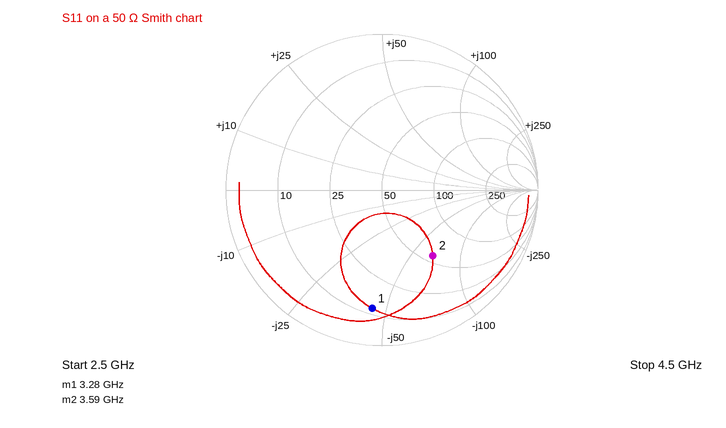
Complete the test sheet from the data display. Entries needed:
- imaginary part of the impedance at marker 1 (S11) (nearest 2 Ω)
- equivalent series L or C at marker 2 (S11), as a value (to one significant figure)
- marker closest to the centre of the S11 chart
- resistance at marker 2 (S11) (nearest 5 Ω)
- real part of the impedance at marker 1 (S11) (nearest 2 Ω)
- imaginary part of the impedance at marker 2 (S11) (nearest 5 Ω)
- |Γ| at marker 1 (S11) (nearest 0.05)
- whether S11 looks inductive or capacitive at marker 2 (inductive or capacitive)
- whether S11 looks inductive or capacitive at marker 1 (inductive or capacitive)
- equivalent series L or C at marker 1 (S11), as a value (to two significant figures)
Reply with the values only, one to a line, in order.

-44 Ω
700 fF
marker 2
55 Ω
12 Ω
-65 Ω
0.75
capacitive
capacitive
1.1 pF
